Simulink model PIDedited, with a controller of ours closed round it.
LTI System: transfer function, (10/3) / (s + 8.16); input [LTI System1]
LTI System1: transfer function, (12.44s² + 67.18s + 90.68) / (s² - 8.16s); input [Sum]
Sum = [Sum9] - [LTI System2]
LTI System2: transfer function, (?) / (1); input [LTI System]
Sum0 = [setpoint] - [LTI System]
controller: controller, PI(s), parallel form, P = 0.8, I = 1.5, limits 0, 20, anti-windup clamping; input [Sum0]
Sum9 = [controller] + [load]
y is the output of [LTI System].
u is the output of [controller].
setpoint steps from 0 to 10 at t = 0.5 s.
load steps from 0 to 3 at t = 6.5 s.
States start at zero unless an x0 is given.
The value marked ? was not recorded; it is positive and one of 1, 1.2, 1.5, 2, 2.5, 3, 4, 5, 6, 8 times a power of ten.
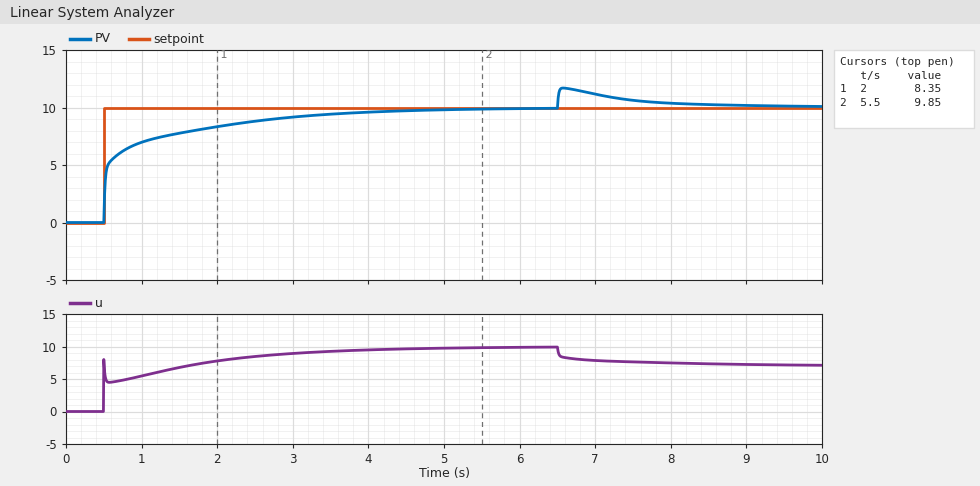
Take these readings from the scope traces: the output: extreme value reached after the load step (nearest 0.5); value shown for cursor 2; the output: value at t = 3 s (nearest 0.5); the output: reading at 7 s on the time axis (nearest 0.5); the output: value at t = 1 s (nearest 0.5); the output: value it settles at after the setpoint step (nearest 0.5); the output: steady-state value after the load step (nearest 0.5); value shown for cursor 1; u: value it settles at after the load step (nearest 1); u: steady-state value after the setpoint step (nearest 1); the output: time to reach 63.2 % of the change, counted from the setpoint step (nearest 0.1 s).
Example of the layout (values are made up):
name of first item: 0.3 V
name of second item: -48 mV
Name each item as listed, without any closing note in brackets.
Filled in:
the output: extreme value reached after the load step: 11.5
value shown for cursor 2: 9.85
the output: value at t = 3 s: 9.0
the output: reading at 7 s on the time axis: 11.0
the output: value at t = 1 s: 7.0
the output: value it settles at after the setpoint step: 10.0
the output: steady-state value after the load step: 10.0
value shown for cursor 1: 8.35
u: value it settles at after the load step: 7
u: steady-state value after the setpoint step: 10
the output: time to reach 63.2 % of the change, counted from the setpoint step: 0.3 s
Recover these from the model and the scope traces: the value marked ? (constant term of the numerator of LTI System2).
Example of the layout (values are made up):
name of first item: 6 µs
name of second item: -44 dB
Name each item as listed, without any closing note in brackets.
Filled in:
the value marked ?: 1
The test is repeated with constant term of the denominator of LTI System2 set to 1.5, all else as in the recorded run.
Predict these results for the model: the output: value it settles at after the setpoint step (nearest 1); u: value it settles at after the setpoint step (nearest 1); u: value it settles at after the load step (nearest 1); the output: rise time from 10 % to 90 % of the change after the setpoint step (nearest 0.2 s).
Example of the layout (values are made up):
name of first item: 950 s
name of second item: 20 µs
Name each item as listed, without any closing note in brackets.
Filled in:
the output: value it settles at after the setpoint step: 10
u: value it settles at after the setpoint step: 7
u: value it settles at after the load step: 4
the output: rise time from 10 % to 90 % of the change after the setpoint step: 1.8 s
